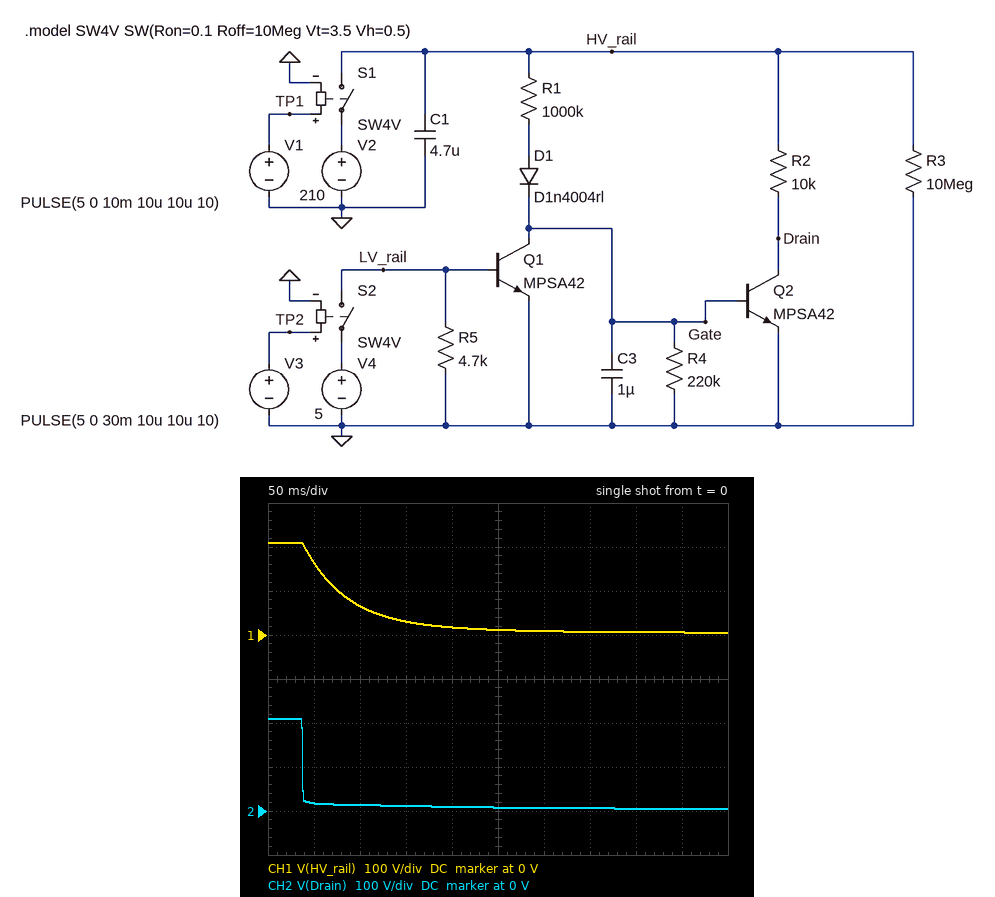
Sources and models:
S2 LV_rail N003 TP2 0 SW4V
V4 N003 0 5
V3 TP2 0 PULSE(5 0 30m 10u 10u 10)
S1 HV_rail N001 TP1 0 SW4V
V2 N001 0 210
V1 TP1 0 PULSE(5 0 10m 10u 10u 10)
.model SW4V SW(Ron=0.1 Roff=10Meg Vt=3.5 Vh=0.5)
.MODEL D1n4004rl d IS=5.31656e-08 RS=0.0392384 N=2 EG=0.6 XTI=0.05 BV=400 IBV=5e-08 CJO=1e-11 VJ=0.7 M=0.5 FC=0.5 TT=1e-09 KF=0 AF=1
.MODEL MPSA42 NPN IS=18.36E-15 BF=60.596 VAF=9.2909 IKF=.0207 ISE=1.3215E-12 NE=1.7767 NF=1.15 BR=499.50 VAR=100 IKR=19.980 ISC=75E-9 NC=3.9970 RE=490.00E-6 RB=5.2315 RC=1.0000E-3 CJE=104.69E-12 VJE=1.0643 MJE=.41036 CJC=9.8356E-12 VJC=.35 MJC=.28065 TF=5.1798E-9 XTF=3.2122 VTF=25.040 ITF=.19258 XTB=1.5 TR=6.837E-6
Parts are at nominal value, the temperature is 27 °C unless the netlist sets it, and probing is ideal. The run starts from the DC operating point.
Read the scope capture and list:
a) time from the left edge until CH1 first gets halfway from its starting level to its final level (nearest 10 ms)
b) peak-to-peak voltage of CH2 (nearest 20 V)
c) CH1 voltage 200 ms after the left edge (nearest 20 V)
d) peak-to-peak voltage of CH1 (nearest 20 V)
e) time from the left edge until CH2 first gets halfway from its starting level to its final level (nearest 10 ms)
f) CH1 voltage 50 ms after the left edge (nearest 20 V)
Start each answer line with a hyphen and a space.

- 70 ms
- 200 V
- 20 V
- 200 V
- 40 ms
- 160 V
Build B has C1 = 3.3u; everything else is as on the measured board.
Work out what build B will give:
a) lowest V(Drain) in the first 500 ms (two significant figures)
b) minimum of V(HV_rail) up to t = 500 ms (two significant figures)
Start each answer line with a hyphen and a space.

- 4.4 V
- 4.6 V
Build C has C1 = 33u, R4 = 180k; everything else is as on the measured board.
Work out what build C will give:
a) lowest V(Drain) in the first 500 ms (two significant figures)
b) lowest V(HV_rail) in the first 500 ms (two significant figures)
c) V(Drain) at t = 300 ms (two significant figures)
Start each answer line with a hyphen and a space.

- 14 V
- 62 V
- 15 V
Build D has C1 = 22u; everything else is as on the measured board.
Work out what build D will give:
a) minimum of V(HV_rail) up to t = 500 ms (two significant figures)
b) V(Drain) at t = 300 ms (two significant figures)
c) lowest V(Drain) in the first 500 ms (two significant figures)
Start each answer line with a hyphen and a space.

- 37 V
- 14 V
- 12 V
